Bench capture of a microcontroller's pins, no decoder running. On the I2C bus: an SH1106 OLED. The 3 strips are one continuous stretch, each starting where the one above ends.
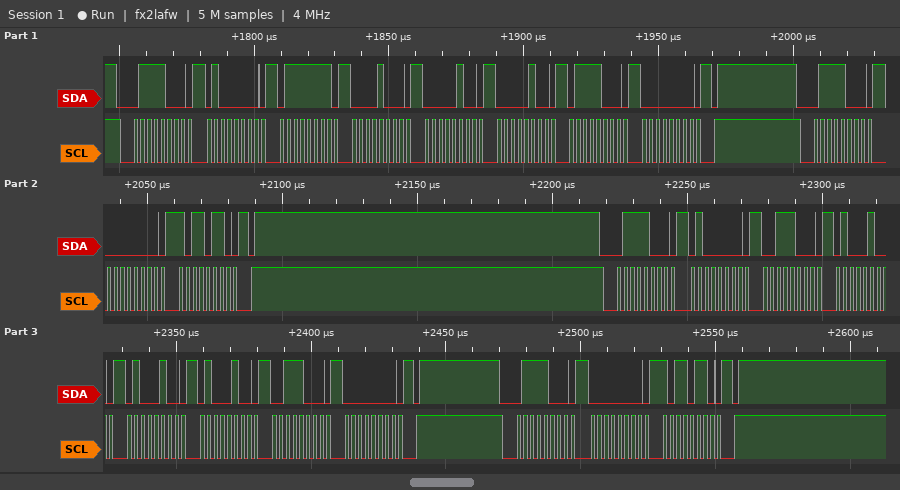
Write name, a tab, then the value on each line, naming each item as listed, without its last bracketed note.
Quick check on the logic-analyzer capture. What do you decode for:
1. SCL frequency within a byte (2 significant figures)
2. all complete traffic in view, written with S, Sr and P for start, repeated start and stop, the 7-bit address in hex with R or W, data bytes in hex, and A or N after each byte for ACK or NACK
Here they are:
SCL frequency within a byte	400 kHz
all complete traffic in view, written with S, Sr and P for start, repeated start and stop, the 7-bit address in hex with R or W, data bytes in hex, and A or N after each byte for ACK or NACK	S 3CW A 40 A 7F A 08 A 04 A 04 A 78 A 00 A P S 3CW A 00 A B6 A P S 3CW A 40 A 38 A 44 A 44 A 44 A 38 A 00 A P S 3CW A 00 A B6 A P
